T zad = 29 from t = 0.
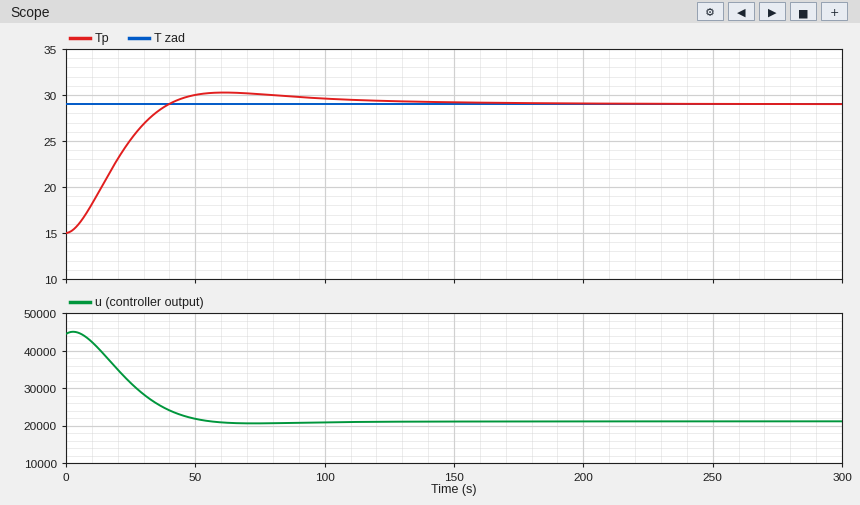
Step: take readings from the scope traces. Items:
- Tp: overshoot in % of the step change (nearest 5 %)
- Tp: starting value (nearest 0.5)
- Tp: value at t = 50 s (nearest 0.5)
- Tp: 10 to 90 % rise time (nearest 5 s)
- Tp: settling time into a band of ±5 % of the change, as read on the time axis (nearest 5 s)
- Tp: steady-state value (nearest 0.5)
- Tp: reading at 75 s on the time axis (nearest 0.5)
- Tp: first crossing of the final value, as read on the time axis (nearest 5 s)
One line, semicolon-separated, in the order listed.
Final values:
10 %; 15.0; 30.0; 25 s; 95 s; 29.0; 30.0; 40 s
